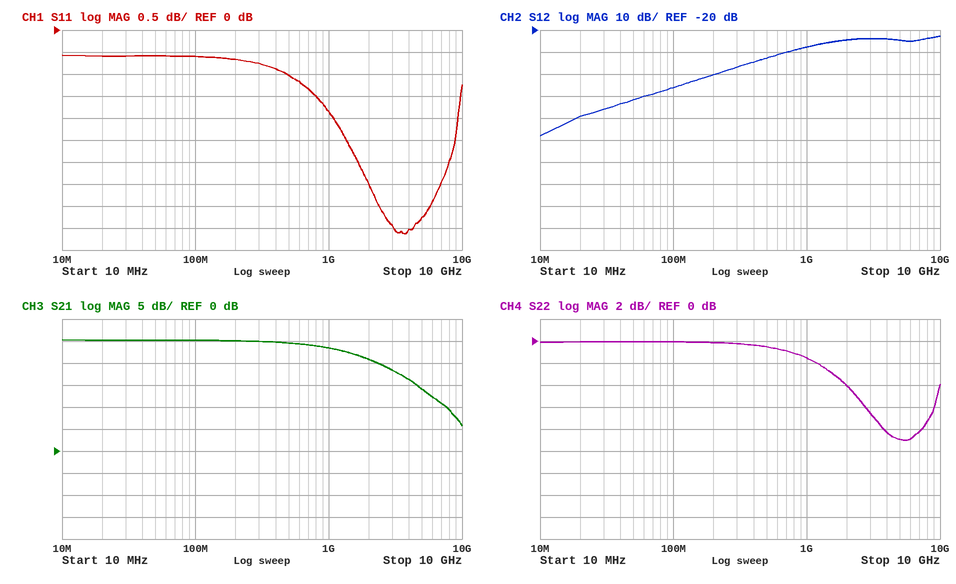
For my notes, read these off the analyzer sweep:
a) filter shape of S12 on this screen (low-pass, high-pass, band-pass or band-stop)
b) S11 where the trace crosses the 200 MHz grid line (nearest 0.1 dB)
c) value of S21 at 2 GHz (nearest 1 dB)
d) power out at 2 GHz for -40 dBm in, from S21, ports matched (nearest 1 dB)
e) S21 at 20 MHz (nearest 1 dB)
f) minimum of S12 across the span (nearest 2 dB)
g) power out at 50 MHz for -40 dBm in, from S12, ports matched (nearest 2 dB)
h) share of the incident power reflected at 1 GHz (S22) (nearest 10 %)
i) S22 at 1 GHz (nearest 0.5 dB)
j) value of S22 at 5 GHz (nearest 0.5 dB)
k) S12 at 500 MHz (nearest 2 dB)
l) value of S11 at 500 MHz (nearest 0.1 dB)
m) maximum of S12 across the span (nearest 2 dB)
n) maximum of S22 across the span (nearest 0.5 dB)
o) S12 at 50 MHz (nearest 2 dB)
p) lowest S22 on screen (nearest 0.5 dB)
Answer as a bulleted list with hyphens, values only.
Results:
- high-pass
- -0.7 dB
- 21 dB
- -19 dBm
- 25 dB
- -68 dB
- -92 dBm
- 70 %
- -1.5 dB
- -9.0 dB
- -32 dB
- -1.0 dB
- -22 dB
- 0.0 dB
- -52 dB
- -9.0 dB
